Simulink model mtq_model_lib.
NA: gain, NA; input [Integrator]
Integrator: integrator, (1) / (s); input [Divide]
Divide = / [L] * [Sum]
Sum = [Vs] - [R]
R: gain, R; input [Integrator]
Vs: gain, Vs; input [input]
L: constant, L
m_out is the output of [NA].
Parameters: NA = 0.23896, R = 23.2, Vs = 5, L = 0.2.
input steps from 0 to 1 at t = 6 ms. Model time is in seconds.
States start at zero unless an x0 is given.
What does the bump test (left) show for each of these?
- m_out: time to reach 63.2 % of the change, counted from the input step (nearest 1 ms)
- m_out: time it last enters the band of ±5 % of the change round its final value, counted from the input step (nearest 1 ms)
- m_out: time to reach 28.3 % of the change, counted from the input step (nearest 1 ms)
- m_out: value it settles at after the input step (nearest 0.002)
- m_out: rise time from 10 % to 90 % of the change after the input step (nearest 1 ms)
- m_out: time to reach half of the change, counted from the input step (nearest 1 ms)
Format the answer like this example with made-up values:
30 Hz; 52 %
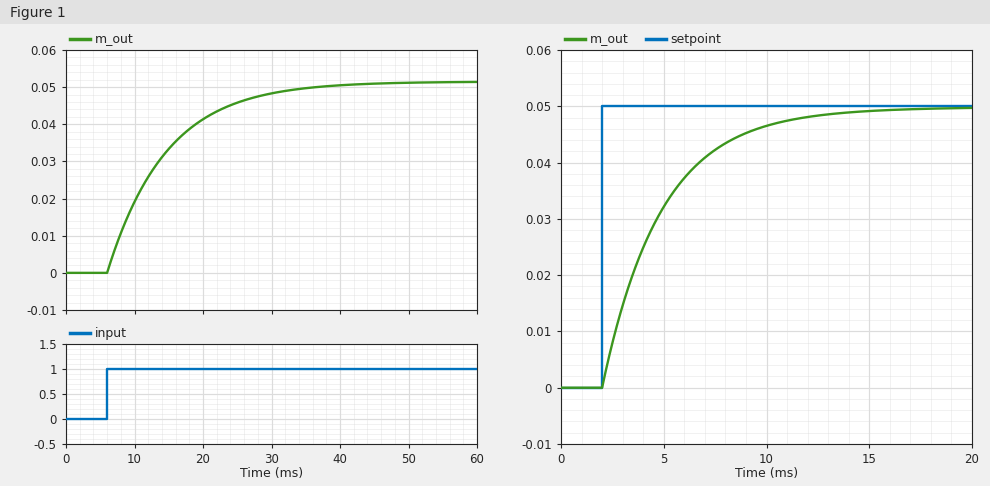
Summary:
9 ms; 26 ms; 3 ms; 0.052; 19 ms; 6 ms
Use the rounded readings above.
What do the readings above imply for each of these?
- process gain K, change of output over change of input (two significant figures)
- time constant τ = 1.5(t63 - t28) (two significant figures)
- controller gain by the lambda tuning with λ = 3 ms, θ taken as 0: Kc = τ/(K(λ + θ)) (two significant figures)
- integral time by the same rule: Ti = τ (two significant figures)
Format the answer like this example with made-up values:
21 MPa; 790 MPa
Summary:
0.052; 9.0 ms; 58; 9.0 ms
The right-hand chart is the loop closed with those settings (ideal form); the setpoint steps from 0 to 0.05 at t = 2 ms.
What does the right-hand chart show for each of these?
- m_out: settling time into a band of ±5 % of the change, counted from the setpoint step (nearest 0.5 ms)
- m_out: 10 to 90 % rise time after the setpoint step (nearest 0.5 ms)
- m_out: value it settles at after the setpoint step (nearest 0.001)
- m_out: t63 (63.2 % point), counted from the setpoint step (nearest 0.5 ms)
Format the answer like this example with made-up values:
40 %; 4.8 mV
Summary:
9.0 ms; 6.5 ms; 0.050; 3.0 ms
